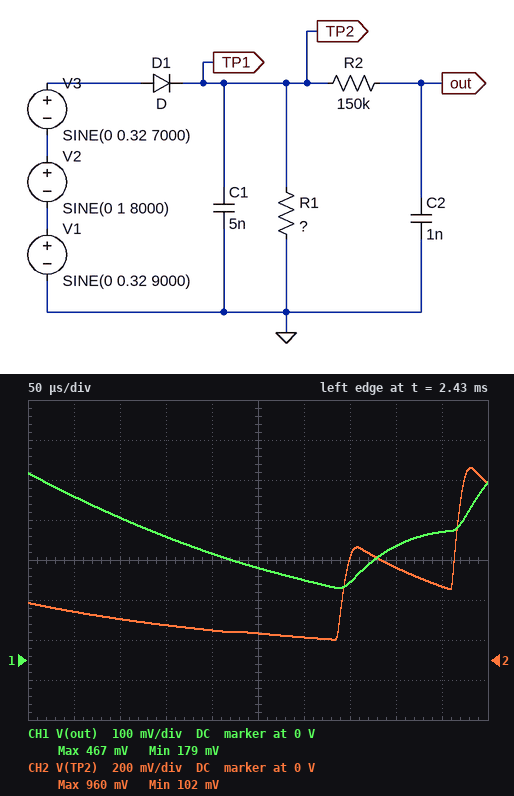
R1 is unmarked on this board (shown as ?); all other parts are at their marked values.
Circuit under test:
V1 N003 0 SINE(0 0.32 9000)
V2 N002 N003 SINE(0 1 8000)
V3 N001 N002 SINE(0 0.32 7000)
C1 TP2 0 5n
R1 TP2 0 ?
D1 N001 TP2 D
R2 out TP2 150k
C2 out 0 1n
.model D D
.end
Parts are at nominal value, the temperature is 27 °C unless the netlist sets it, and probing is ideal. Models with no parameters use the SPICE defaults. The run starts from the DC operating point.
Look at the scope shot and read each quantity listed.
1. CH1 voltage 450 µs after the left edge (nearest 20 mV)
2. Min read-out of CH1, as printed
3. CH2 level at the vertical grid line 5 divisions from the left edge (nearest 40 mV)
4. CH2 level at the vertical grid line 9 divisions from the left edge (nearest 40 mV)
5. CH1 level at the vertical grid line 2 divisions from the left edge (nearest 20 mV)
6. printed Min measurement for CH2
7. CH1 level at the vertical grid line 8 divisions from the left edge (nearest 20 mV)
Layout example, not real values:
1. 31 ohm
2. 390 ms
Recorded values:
1. 320 mV
2. 179 mV
3. 120 mV
4. 360 mV
5. 360 mV
6. 102 mV
7. 280 mV
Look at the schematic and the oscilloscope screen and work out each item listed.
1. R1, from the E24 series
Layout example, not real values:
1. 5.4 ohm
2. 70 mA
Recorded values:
1. 47 kΩ
